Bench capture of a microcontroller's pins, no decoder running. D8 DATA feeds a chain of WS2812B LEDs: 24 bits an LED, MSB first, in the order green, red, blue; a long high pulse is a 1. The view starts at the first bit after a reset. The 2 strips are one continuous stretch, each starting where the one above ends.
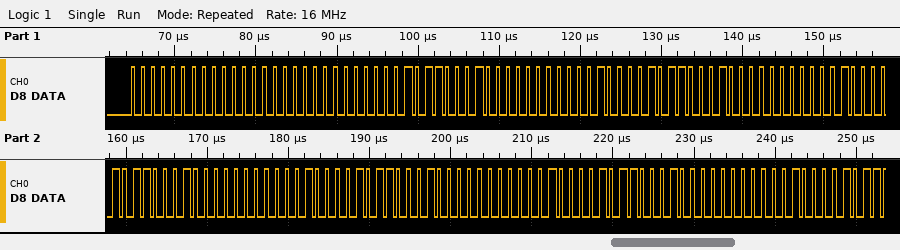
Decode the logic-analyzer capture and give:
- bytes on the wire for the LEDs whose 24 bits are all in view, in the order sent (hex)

00 00 00 16 20 02 16 20 02 16 20 02 16 20 02 16 20 02
